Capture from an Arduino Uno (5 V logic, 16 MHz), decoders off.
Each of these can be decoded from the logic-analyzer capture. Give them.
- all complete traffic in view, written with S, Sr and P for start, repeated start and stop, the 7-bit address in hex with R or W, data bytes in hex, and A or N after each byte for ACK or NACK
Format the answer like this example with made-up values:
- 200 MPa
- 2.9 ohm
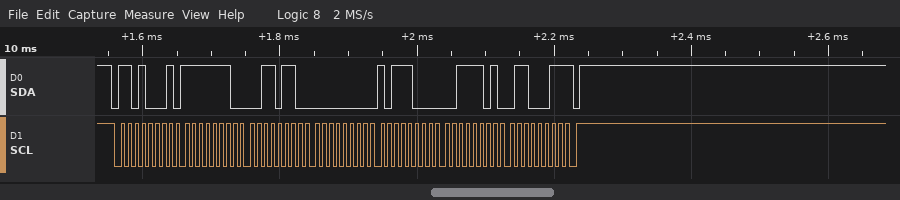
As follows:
- S 68R A FE A 36 A 00 A B8 A 3D A 63 N P
